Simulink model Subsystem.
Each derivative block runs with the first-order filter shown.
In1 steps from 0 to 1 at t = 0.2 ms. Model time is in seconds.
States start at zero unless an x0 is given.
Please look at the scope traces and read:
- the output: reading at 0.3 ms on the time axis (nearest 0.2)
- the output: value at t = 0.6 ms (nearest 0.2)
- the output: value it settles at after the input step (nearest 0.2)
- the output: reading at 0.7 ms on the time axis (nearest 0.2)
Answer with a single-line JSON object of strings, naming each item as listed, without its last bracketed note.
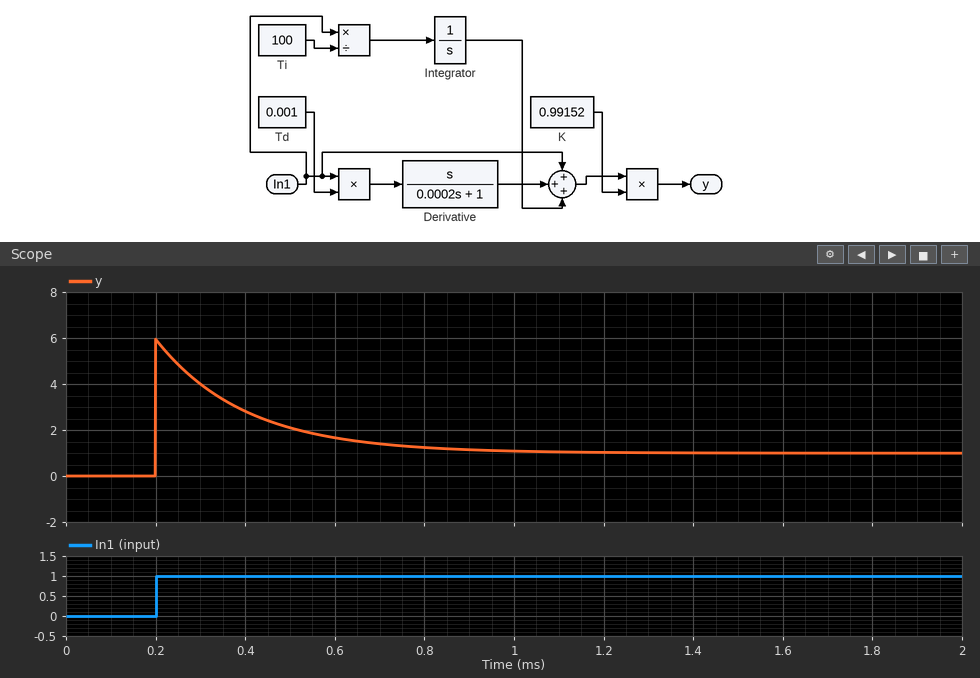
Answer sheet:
{"the output: reading at 0.3 ms on the time axis": "4.0", "the output: value at t = 0.6 ms": "1.6", "the output: value it settles at after the input step": "1.0", "the output: reading at 0.7 ms on the time axis": "1.4"}
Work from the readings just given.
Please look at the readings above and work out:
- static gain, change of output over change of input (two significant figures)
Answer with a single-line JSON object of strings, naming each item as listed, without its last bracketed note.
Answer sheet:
{"static gain, change of output over change of input": "1.0"}
